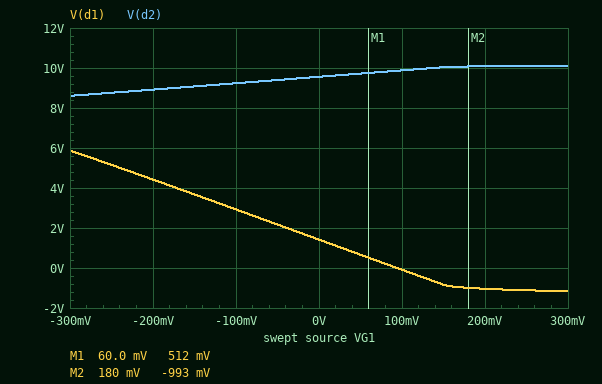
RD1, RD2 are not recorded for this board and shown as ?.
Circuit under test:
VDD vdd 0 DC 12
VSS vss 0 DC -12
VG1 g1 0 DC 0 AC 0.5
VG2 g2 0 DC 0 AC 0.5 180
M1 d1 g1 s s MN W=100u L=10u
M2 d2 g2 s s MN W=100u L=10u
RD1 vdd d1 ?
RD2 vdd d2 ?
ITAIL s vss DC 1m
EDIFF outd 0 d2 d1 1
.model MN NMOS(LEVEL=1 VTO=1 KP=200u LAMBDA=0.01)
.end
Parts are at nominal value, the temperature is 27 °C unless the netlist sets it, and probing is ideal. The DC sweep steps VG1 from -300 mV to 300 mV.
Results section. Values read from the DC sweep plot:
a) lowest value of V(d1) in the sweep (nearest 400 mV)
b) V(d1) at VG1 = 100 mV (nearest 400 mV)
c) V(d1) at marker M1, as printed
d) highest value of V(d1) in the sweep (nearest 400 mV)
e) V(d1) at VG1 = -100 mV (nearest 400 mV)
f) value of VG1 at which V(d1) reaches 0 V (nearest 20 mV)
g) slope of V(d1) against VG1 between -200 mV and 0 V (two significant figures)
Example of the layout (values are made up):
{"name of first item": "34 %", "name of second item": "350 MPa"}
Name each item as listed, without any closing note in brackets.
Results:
{"lowest value of V(d1) in the sweep": "-1.2 V", "V(d1) at VG1 = 100 mV": "0 V", "V(d1) at marker M1, as printed": "512 mV", "highest value of V(d1) in the sweep": "6.0 V", "V(d1) at VG1 = -100 mV": "2.8 V", "value of VG1 at which V(d1) reaches 0 V": "100 mV", "slope of V(d1) against VG1 between -200 mV and 0 V": "-15 V/V"}
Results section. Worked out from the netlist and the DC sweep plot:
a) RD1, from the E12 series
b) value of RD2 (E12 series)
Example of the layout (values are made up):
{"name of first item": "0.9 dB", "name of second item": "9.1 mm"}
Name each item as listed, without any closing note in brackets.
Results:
{"RD1, from the E12 series": "22 kΩ", "value of RD2": "4.7 kΩ"}
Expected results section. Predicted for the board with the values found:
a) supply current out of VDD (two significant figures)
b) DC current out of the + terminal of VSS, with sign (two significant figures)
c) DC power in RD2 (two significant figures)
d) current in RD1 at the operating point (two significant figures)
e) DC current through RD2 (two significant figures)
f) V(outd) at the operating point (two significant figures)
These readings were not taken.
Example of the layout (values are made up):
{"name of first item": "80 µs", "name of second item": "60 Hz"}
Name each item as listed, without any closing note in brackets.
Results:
{"supply current out of VDD": "1.0 mA", "DC current out of the + terminal of VSS, with sign": "-1.0 mA", "DC power in RD2": "1.3 mW", "current in RD1 at the operating point": "480 µA", "DC current through RD2": "520 µA", "V(outd) at the operating point": "8.1 V"}
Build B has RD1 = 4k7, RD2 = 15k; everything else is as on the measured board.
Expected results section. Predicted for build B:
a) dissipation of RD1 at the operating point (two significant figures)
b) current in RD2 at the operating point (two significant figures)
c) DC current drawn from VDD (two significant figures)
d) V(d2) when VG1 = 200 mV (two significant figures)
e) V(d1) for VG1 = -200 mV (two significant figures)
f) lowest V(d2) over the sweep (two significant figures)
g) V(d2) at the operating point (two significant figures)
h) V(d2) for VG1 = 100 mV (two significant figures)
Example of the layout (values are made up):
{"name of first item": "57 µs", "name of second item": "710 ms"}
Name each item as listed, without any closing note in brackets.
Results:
{"dissipation of RD1 at the operating point": "1.2 mW", "current in RD2 at the operating point": "490 µA", "DC current drawn from VDD": "1.0 mA", "V(d2) when VG1 = 200 mV": "6.8 V", "V(d1) for VG1 = -200 mV": "10 V", "lowest V(d2) over the sweep": "1.6 V", "V(d2) at the operating point": "4.7 V", "V(d2) for VG1 = 100 mV": "5.7 V"}
